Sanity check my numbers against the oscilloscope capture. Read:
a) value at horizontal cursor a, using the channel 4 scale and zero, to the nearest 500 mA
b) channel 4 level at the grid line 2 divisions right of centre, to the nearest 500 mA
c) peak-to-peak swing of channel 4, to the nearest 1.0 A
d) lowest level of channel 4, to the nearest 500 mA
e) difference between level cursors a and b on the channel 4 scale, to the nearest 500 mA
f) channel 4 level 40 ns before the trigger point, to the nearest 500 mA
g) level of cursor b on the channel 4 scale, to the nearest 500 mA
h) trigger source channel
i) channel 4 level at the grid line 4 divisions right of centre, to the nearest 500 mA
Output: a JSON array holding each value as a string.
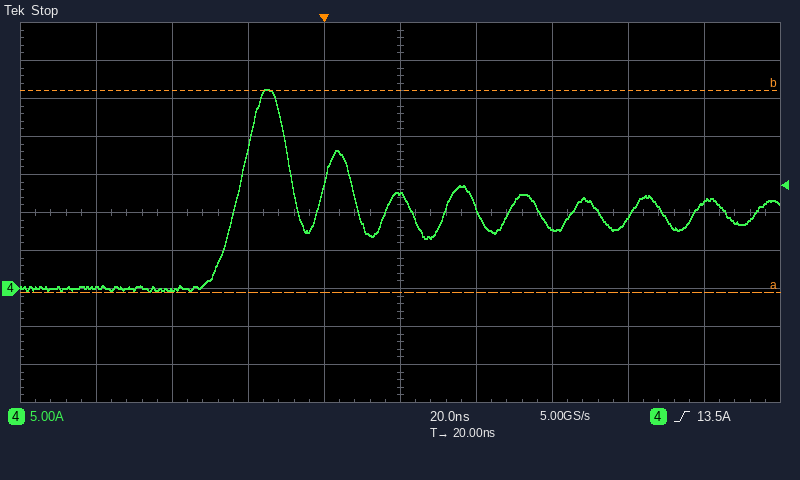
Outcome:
["-500 mA", "8.0 A", "27.0 A", "-500 mA", "26.5 A", "0.0 A", "26.0 A", "channel 4", "11.5 A"]
